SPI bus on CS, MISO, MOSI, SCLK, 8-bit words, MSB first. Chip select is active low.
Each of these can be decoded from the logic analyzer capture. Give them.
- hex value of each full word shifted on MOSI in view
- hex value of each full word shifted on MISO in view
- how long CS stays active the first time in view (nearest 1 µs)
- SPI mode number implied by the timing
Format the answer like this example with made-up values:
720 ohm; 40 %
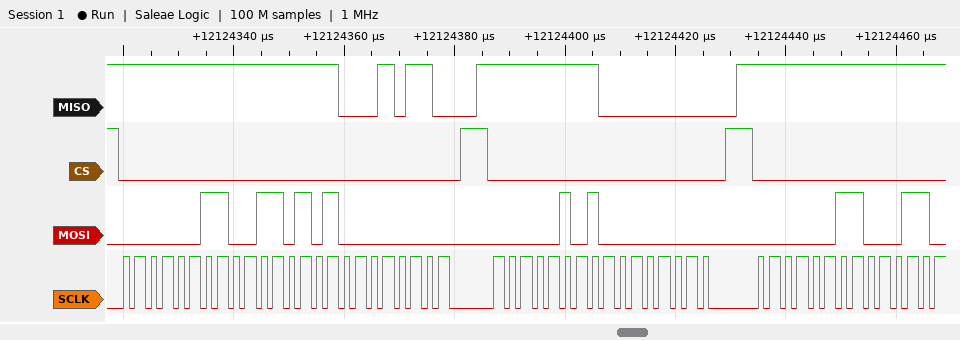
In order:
03, 35, 00, 05, 00, 03; FF, FF, 16, FF, 00, FF; 62 µs; 0
